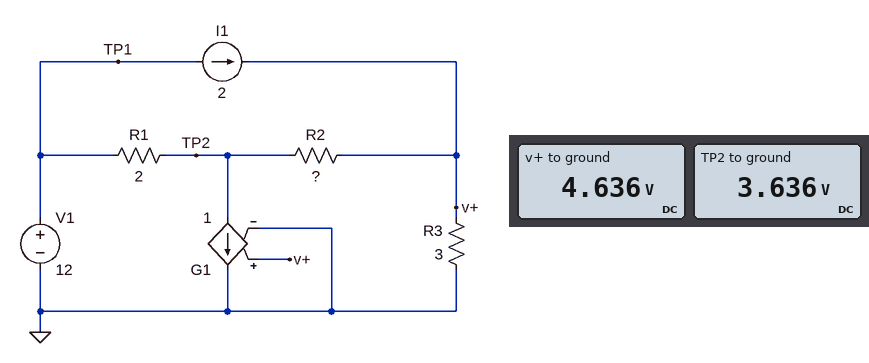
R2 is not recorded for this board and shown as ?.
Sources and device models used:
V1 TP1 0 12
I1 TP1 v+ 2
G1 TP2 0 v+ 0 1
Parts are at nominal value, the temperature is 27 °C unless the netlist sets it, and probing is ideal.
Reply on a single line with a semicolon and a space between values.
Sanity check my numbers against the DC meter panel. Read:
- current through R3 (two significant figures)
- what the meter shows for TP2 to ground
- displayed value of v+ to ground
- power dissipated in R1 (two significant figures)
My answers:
1.5 A; 3.636 V; 4.636 V; 35 W
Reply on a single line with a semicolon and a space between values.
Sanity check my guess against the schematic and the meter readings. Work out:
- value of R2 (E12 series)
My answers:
2.2 Ω
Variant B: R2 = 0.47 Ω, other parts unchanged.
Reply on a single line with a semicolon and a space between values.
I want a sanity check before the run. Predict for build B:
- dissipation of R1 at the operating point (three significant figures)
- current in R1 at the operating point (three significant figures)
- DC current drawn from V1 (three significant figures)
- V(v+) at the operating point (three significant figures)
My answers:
30.5 W; 3.91 A; 5.91 A; 4.43 V
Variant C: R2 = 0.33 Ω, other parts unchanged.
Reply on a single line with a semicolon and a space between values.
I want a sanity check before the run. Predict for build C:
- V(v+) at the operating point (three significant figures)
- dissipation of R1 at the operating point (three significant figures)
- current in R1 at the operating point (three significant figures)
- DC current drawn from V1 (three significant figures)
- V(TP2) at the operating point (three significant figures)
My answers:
4.41 V; 30.1 W; 3.88 A; 5.88 A; 4.24 V
